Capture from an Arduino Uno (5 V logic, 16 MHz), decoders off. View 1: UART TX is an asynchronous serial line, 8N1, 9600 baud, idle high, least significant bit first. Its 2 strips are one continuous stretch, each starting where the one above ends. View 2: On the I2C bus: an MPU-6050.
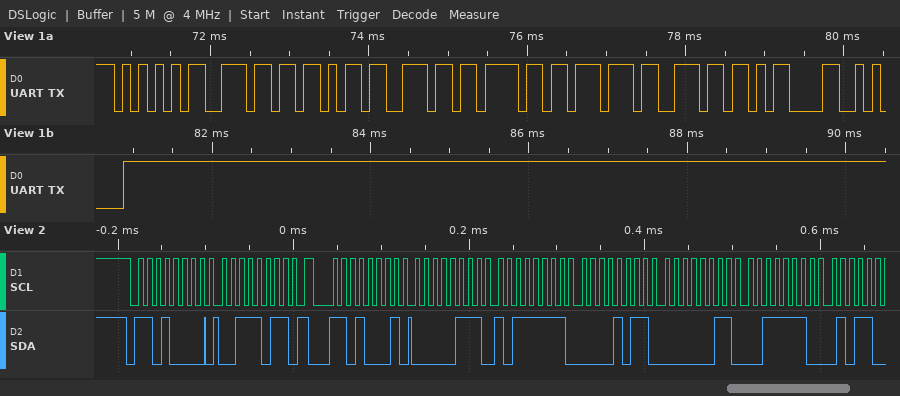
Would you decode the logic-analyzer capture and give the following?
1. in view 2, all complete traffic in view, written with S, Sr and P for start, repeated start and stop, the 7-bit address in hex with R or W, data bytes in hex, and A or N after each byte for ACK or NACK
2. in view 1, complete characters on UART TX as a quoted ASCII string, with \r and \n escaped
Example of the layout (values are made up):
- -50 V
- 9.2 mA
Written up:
- S 68W A 3B A Sr 68R A 07 A BF A 0B A 03 A 3E A
- "Unknown\r\n"
